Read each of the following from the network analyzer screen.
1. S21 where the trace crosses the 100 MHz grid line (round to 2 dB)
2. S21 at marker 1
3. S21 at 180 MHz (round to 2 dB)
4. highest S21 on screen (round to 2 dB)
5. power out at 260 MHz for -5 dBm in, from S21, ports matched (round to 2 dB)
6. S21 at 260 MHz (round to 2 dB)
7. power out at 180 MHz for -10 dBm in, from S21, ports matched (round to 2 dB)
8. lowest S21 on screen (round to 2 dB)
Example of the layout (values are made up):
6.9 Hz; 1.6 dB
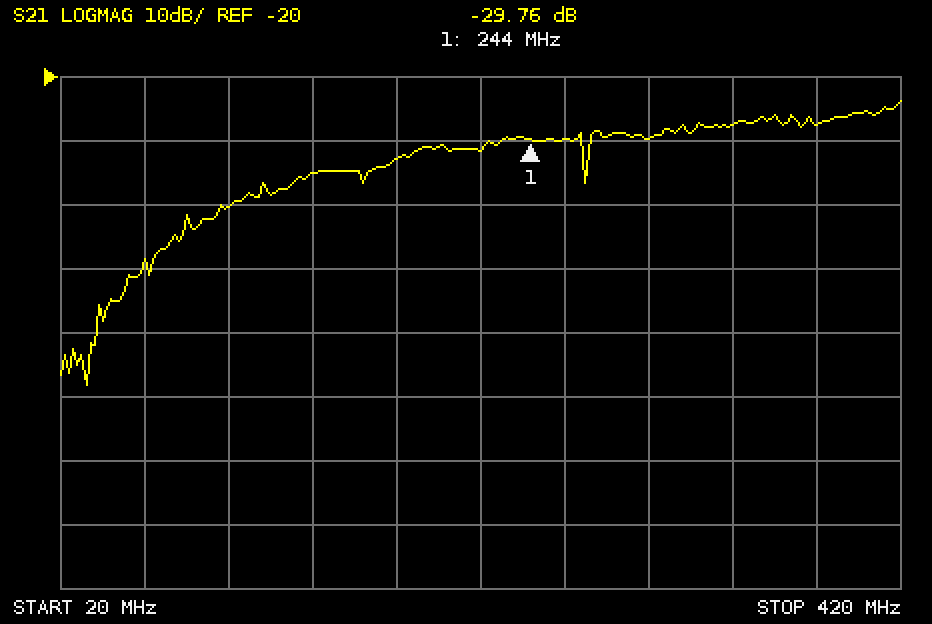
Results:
-40 dB; -29.76 dB; -32 dB; -24 dB; -34 dBm; -30 dB; -42 dBm; -68 dB
